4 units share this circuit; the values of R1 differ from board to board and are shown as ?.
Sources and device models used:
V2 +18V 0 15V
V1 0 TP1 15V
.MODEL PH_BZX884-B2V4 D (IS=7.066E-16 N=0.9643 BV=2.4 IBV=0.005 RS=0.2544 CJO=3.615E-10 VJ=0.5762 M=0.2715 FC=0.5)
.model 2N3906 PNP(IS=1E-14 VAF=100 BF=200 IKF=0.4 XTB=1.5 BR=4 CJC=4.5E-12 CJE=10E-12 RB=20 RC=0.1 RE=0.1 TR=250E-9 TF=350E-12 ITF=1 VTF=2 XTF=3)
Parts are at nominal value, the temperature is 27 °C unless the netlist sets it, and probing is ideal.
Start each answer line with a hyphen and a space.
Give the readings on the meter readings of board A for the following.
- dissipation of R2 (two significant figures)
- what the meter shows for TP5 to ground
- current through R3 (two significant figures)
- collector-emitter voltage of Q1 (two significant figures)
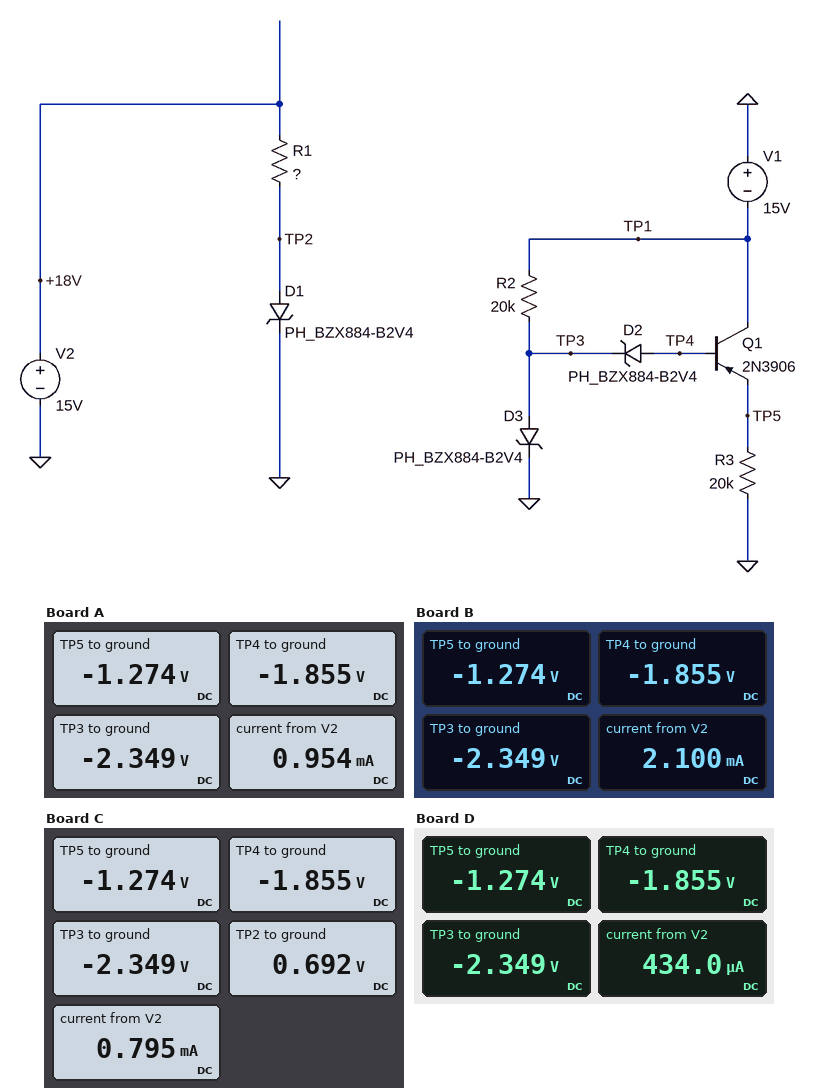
- 8.0 mW
- -1.274 V
- 64 µA
- -14 V
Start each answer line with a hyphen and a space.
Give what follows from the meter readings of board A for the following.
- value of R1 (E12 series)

- 15 kΩ
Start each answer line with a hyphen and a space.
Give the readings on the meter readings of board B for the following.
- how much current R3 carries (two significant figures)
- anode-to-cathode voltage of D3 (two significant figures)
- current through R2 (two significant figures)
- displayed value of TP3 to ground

- 64 µA
- -2.3 V
- 630 µA
- -2.349 V
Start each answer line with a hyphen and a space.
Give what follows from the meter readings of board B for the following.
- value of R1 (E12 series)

- 6.8 kΩ
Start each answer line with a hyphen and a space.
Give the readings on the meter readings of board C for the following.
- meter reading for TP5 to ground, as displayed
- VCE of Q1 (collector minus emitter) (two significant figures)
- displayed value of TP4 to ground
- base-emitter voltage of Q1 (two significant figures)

- -1.274 V
- -14 V
- -1.855 V
- -580 mV
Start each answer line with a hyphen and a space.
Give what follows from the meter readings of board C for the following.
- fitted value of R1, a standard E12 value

- 18 kΩ
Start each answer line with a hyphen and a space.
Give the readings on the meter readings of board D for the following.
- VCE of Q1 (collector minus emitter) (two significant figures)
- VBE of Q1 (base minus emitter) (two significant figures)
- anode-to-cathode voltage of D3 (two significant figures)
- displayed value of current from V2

- -14 V
- -580 mV
- -2.3 V
- 434.0 µA
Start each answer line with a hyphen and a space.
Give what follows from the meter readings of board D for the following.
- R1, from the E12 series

- 33 kΩ
